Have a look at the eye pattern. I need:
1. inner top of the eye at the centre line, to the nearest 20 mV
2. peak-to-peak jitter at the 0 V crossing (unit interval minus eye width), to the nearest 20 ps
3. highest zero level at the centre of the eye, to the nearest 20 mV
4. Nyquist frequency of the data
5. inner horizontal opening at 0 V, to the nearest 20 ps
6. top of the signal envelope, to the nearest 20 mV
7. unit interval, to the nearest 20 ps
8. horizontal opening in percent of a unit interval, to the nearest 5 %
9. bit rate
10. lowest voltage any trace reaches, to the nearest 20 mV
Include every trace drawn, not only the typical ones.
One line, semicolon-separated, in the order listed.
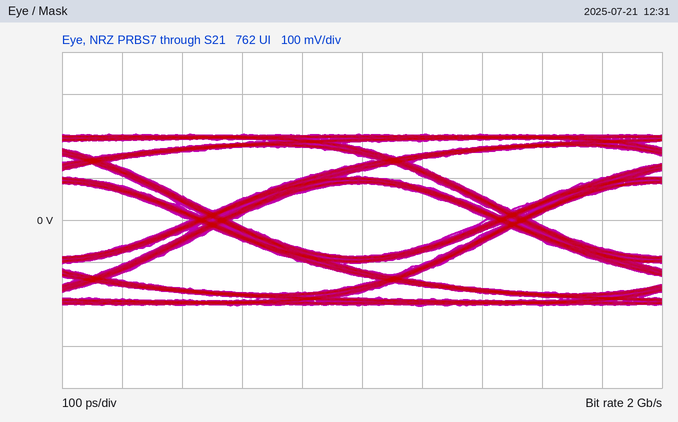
80 mV; 80 ps; -80 mV; 1 GHz; 420 ps; 200 mV; 500 ps; 85 %; 2 Gb/s; -200 mV
